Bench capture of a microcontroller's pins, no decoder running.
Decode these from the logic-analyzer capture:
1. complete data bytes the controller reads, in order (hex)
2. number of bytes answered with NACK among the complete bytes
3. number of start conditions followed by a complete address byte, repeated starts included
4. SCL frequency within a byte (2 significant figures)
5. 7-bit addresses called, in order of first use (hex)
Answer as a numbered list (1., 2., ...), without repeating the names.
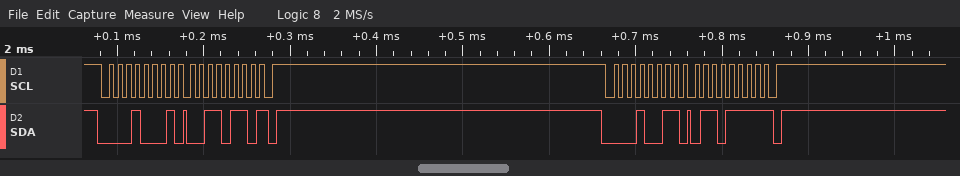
1. 36 6F
2. 2
3. 2
4. 100 kHz
5. 0x08 0x09
